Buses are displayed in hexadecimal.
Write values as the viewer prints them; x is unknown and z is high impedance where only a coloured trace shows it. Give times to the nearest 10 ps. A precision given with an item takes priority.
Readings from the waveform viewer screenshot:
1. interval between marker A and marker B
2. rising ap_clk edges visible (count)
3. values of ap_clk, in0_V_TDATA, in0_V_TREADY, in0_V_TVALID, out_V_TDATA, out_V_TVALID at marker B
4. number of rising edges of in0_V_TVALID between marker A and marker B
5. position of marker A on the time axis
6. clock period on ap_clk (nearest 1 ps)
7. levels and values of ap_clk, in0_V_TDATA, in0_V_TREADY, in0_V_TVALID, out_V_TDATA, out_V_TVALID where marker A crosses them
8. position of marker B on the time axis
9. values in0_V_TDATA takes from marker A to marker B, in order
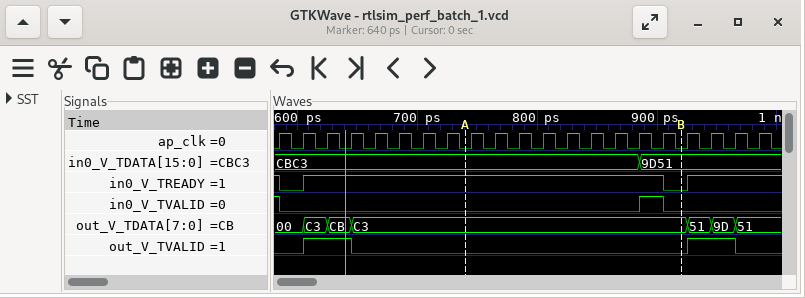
180 ps
21
ap_clk=0, in0_V_TDATA=9D51, in0_V_TREADY=0, in0_V_TVALID=0, out_V_TDATA=C3, out_V_TVALID=0
1
740 ps
20 ps
ap_clk=0, in0_V_TDATA=CBC3, in0_V_TREADY=1, in0_V_TVALID=0, out_V_TDATA=C3, out_V_TVALID=0
920 ps
CBC3, 9D51
